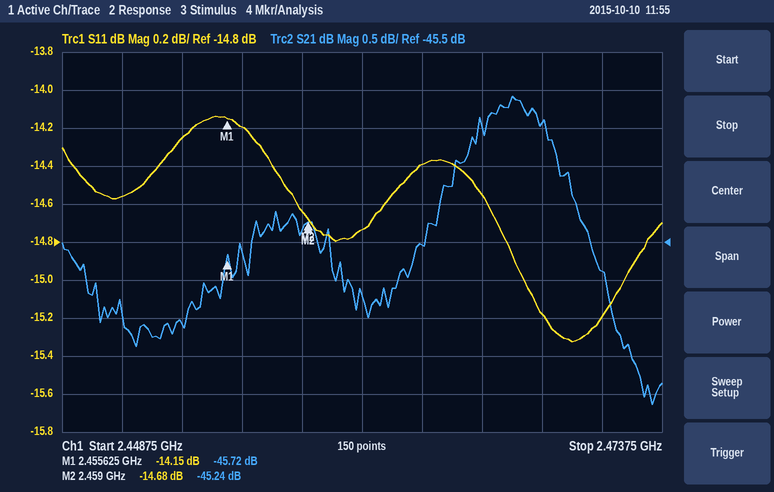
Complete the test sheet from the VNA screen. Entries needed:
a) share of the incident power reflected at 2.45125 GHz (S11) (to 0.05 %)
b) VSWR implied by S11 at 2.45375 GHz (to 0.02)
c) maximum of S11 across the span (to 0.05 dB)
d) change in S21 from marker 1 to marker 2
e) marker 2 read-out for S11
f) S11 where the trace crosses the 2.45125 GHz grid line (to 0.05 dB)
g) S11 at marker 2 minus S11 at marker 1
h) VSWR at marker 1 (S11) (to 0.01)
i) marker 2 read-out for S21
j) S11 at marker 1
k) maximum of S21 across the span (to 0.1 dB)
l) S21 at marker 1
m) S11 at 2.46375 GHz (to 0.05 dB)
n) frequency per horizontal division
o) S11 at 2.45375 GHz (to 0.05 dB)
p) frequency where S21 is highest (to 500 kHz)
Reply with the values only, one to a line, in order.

3.50 %
1.48
-14.15 dB
0.48 dB
-14.68 dB
-14.55 dB
-0.53 dB
1.49
-45.24 dB
-14.15 dB
-43.6 dB
-45.72 dB
-14.40 dB
2.5 MHz
-14.25 dB
2.4675 GHz
